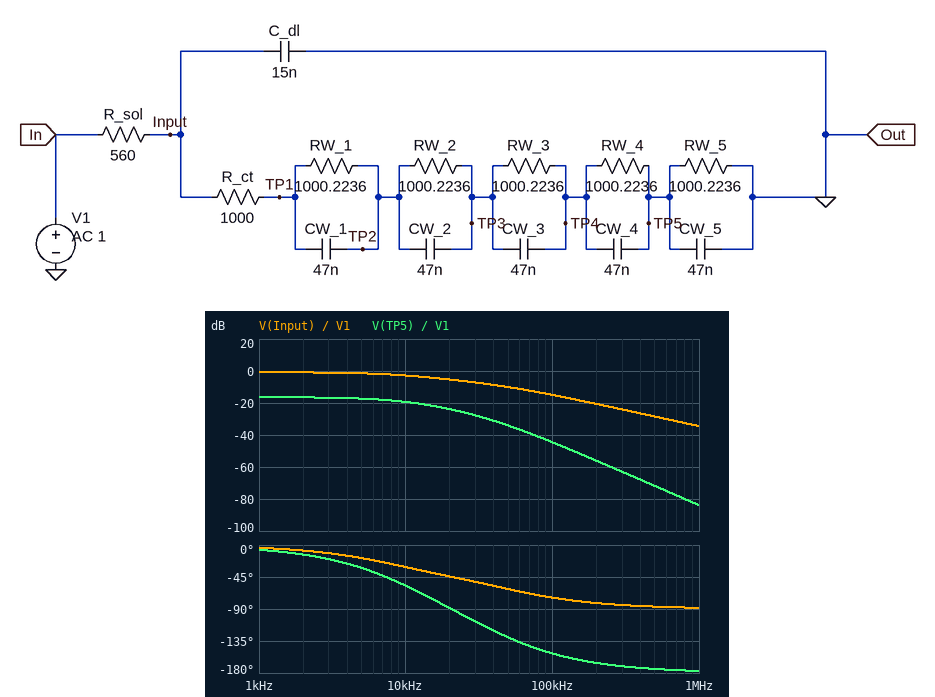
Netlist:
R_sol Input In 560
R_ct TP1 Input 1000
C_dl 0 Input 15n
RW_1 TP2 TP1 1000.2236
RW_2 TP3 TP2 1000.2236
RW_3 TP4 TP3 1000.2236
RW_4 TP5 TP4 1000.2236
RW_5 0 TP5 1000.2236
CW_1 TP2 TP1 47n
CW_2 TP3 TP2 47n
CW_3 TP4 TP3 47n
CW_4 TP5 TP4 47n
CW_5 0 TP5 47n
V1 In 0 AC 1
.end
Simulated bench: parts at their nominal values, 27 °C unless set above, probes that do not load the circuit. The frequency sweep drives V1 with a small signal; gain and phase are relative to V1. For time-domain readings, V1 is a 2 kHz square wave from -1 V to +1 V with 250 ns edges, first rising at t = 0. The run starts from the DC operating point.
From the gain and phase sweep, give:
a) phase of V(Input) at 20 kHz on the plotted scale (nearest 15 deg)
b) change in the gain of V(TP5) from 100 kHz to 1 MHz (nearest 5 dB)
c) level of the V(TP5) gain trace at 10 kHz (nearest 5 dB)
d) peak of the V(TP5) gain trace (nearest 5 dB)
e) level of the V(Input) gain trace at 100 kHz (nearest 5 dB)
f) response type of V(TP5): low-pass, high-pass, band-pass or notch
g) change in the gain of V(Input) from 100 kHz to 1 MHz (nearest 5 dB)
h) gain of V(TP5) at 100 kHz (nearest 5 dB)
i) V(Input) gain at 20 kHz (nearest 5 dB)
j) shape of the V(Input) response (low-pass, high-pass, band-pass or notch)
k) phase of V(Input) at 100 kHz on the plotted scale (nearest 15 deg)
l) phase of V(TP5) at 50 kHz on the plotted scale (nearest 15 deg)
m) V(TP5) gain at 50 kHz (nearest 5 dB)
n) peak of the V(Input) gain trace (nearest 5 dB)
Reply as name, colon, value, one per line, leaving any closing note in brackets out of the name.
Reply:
phase of V(Input) at 20 kHz on the plotted scale: -45 deg
change in the gain of V(TP5) from 100 kHz to 1 MHz: -40 dB
level of the V(TP5) gain trace at 10 kHz: -20 dB
peak of the V(TP5) gain trace: -15 dB
level of the V(Input) gain trace at 100 kHz: -15 dB
response type of V(TP5): low-pass, high-pass, band-pass or notch: low-pass
change in the gain of V(Input) from 100 kHz to 1 MHz: -20 dB
gain of V(TP5) at 100 kHz: -45 dB
V(Input) gain at 20 kHz: -5 dB
shape of the V(Input) response: low-pass
phase of V(Input) at 100 kHz on the plotted scale: -75 deg
phase of V(TP5) at 50 kHz on the plotted scale: -135 deg
V(TP5) gain at 50 kHz: -35 dB
peak of the V(Input) gain trace: 0 dB
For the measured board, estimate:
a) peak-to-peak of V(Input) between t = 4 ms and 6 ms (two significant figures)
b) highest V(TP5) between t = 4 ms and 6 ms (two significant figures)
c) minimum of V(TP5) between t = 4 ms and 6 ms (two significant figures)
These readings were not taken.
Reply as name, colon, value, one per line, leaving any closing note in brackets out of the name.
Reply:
peak-to-peak of V(Input) between t = 4 ms and 6 ms: 1.8 V
highest V(TP5) between t = 4 ms and 6 ms: 150 mV
minimum of V(TP5) between t = 4 ms and 6 ms: -150 mV
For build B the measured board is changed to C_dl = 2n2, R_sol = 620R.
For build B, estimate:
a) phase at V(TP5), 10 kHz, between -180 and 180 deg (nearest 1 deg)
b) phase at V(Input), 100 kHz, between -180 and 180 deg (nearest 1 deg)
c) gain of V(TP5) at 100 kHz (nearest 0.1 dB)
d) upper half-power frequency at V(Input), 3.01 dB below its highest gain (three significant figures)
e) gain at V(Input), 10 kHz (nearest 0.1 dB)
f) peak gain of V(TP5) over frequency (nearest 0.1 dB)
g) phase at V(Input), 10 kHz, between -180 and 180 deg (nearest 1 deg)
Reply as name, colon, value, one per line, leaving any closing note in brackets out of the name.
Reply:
phase at V(TP5), 10 kHz, between -180 and 180 deg: -40 deg
phase at V(Input), 100 kHz, between -180 and 180 deg: -31 deg
gain of V(TP5) at 100 kHz: -35.0 dB
upper half-power frequency at V(Input), 3.01 dB below its highest gain: 32.4 kHz
gain at V(Input), 10 kHz: -1.9 dB
peak gain of V(TP5) over frequency: -16.4 dB
phase at V(Input), 10 kHz, between -180 and 180 deg: -14 deg
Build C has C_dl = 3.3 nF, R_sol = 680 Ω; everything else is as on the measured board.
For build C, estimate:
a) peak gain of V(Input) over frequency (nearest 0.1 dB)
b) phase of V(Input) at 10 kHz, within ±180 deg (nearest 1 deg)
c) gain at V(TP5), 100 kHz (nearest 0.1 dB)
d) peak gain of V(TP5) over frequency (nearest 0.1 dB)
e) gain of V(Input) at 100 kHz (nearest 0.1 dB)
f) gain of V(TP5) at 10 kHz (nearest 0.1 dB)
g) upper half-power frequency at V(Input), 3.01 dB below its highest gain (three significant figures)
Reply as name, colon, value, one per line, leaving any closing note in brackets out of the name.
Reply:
peak gain of V(Input) over frequency: -0.9 dB
phase of V(Input) at 10 kHz, within ±180 deg: -17 deg
gain at V(TP5), 100 kHz: -36.6 dB
peak gain of V(TP5) over frequency: -16.5 dB
gain of V(Input) at 100 kHz: -7.0 dB
gain of V(TP5) at 10 kHz: -18.6 dB
upper half-power frequency at V(Input), 3.01 dB below its highest gain: 24.3 kHz
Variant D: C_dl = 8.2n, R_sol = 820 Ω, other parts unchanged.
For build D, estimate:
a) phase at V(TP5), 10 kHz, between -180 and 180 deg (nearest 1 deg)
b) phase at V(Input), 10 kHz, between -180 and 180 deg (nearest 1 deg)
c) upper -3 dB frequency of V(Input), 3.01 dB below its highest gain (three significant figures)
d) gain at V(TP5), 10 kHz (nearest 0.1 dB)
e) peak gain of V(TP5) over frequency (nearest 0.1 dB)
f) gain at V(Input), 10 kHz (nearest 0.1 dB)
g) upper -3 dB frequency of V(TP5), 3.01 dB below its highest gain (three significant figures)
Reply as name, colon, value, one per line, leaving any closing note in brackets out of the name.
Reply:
phase at V(TP5), 10 kHz, between -180 and 180 deg: -55 deg
phase at V(Input), 10 kHz, between -180 and 180 deg: -29 deg
upper -3 dB frequency of V(Input), 3.01 dB below its highest gain: 13.4 kHz
gain at V(TP5), 10 kHz: -19.7 dB
peak gain of V(TP5) over frequency: -16.7 dB
gain at V(Input), 10 kHz: -3.2 dB
upper -3 dB frequency of V(TP5), 3.01 dB below its highest gain: 9.94 kHz
